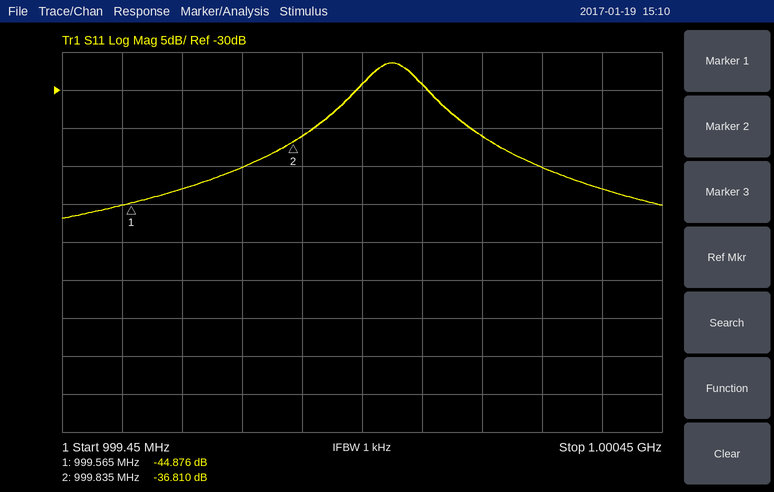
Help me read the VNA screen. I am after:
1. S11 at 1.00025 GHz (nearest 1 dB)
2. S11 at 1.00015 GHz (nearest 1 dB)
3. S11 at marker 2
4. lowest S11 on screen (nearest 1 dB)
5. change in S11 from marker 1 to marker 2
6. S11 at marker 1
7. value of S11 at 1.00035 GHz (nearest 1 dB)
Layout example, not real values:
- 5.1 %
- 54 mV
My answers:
- -40 dB
- -36 dB
- -36.810 dB
- -47 dB
- 8.066 dB
- -44.876 dB
- -43 dB
